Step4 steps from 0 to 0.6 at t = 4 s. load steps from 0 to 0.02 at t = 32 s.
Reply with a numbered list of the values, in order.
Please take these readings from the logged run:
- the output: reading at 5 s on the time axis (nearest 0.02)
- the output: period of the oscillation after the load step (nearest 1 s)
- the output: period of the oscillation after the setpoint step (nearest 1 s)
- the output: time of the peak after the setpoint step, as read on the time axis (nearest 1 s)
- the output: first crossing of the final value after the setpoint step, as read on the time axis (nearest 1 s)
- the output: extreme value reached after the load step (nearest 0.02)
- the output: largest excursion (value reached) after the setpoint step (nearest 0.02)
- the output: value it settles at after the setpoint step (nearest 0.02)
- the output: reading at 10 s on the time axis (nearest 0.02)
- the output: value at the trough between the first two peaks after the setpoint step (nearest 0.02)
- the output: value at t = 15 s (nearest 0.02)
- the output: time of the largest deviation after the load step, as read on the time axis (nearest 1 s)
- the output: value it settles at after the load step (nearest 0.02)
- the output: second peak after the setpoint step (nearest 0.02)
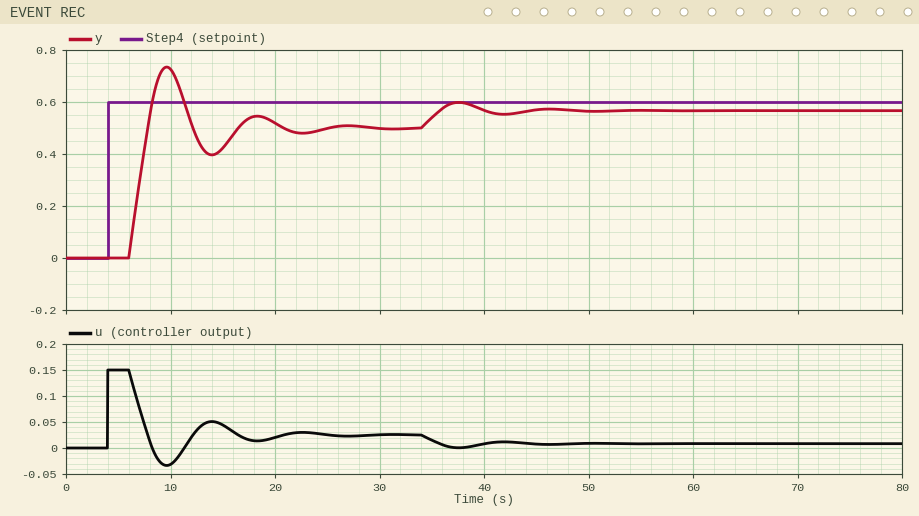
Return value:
1. 0.00
2. 9 s
3. 9 s
4. 10 s
5. 8 s
6. 0.60
7. 0.74
8. 0.50
9. 0.72
10. 0.40
11. 0.42
12. 38 s
13. 0.56
14. 0.54
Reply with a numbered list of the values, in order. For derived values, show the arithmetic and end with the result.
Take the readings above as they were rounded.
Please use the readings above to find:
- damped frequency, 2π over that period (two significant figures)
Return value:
1. 2π / 9 = 0.70 rad/s
